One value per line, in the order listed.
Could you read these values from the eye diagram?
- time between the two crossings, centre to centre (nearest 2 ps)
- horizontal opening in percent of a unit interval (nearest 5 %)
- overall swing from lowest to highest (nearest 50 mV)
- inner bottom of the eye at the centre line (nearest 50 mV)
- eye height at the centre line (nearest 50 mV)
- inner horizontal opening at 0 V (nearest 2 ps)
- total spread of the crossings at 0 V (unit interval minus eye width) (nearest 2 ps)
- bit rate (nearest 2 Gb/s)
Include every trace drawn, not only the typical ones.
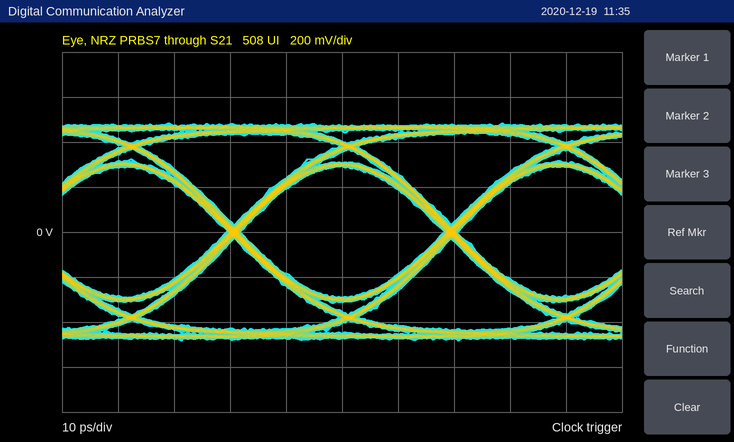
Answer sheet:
38 ps
95 %
950 mV
-300 mV
600 mV
36 ps
2 ps
26 Gb/s
